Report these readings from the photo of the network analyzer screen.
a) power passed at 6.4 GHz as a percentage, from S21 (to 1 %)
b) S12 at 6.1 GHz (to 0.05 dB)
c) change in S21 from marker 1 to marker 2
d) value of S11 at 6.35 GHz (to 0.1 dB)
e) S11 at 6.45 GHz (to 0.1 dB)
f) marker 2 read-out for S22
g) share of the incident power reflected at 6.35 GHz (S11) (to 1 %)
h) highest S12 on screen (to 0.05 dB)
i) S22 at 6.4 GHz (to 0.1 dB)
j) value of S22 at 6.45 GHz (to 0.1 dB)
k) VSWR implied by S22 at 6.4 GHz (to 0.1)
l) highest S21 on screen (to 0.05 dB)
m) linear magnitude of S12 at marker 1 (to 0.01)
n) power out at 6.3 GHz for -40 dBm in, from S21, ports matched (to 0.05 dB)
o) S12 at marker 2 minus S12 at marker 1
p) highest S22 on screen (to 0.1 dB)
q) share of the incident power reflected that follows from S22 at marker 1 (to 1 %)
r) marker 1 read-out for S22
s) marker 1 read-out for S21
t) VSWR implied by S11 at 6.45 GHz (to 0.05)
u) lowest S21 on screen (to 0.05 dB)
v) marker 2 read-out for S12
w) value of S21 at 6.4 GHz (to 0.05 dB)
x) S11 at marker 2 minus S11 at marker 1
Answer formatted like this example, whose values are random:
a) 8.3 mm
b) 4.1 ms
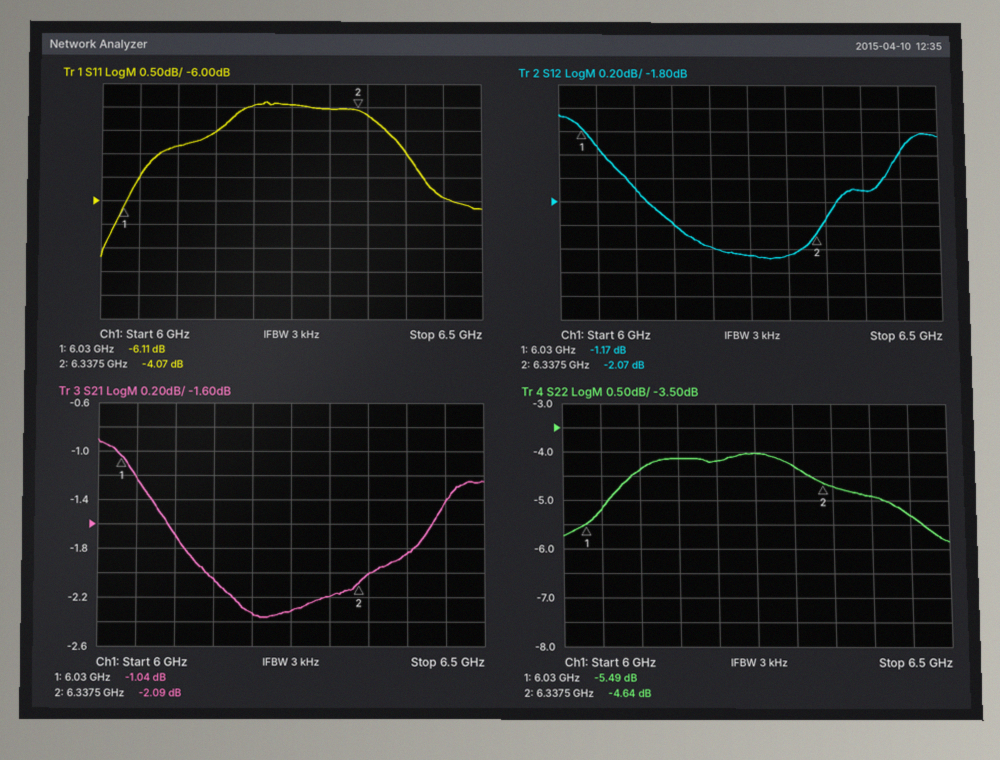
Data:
a) 65 %
b) -1.70 dB
c) -1.05 dB
d) -4.2 dB
e) -5.9 dB
f) -4.64 dB
g) 38 %
h) -1.05 dB
i) -4.9 dB
j) -5.3 dB
k) 3.6
l) -0.90 dB
m) 0.87
n) -42.20 dBm
o) -0.90 dB
p) -4.0 dB
q) 28 %
r) -5.49 dB
s) -1.04 dB
t) 3.05
u) -2.35 dB
v) -2.07 dB
w) -1.85 dB
x) 2.04 dB
